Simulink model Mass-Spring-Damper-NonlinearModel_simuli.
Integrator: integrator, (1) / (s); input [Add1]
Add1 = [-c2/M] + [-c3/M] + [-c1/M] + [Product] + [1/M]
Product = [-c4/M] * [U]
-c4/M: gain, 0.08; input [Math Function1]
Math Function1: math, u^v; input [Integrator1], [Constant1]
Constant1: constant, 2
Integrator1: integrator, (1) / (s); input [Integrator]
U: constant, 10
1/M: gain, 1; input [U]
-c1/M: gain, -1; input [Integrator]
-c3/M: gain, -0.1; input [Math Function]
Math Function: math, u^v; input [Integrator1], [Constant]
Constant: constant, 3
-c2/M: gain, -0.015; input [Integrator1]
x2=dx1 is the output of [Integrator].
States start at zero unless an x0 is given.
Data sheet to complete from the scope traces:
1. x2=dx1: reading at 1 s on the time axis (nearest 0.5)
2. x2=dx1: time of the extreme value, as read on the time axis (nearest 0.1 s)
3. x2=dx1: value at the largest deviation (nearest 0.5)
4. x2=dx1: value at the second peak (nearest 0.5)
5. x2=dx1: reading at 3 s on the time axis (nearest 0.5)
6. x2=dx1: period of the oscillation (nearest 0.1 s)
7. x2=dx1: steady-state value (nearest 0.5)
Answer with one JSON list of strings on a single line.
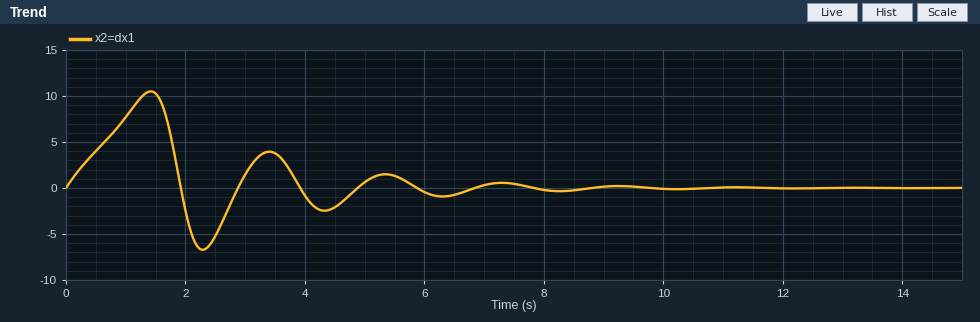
["7.5", "1.4 s", "10.5", "4.0", "1.5", "2.0 s", "0.0"]
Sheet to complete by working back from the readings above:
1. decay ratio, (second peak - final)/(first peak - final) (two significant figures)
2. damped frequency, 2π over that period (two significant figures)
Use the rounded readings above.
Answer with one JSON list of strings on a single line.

["0.38", "3.1 rad/s"]
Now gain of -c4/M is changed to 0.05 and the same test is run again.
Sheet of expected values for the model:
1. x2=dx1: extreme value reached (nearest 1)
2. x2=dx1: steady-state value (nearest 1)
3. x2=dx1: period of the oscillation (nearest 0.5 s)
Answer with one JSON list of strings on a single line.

["8", "0", "2.5 s"]
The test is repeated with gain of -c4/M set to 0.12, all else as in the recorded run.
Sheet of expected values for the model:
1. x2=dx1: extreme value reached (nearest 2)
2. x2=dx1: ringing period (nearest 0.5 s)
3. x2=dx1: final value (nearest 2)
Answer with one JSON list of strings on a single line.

["18", "1.5 s", "0"]
